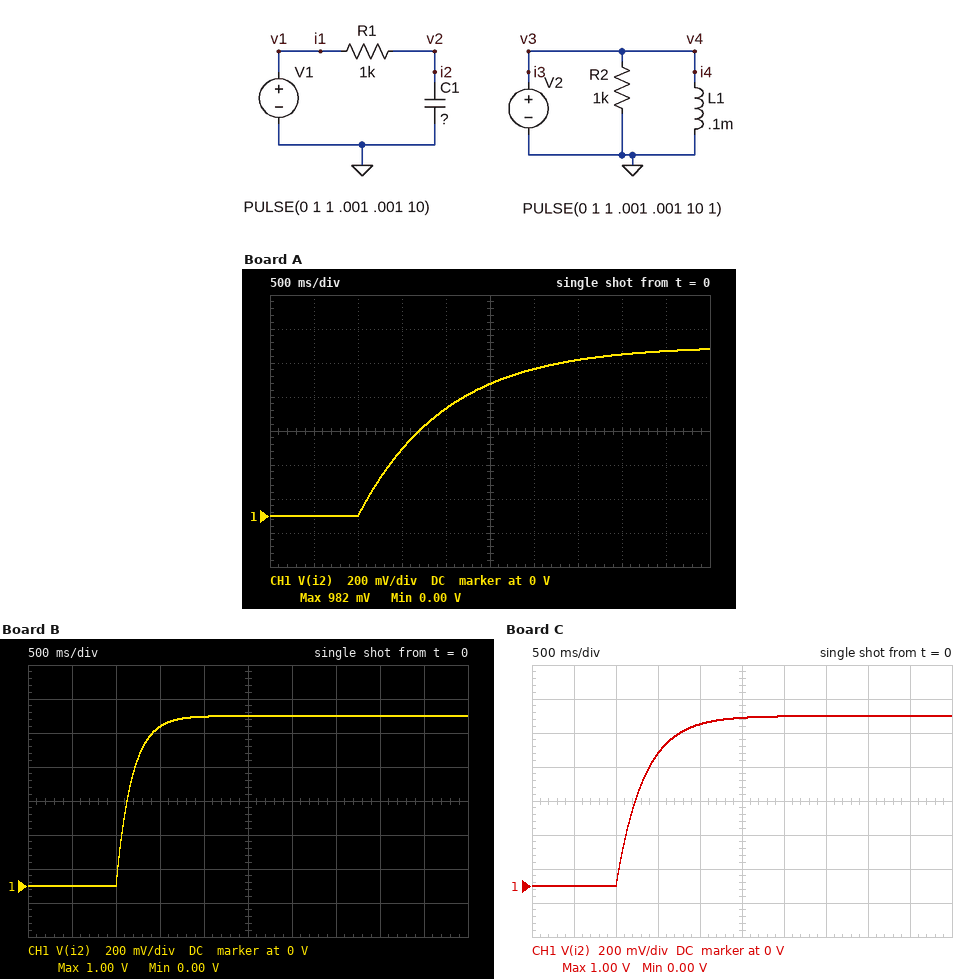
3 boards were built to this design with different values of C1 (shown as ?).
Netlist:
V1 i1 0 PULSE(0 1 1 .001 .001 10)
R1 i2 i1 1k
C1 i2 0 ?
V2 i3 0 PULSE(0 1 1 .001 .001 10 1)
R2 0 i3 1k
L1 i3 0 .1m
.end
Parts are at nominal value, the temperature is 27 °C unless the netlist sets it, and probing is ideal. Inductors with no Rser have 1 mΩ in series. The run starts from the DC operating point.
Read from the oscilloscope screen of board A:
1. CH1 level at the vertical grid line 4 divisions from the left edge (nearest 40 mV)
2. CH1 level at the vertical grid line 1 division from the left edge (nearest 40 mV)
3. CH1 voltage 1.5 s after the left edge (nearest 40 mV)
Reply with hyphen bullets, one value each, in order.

- 640 mV
- 0 V
- 400 mV
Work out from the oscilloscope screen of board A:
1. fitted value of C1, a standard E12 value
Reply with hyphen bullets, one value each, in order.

- 1 mF
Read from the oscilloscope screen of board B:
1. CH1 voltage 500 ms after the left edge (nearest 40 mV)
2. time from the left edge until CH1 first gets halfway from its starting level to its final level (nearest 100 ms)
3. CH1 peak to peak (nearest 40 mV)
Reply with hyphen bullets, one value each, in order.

- 0 V
- 1.1 s
- 1.00 V
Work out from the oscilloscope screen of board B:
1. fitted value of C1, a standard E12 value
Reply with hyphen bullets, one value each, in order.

- 180 µF
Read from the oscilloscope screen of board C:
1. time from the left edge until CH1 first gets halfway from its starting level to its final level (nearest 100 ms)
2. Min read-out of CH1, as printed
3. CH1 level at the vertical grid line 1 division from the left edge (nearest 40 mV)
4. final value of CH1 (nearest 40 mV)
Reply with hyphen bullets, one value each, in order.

- 1.2 s
- 0.00 V
- 0 V
- 1.00 V
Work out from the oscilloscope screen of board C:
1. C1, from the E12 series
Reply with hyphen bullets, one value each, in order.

- 330 µF
